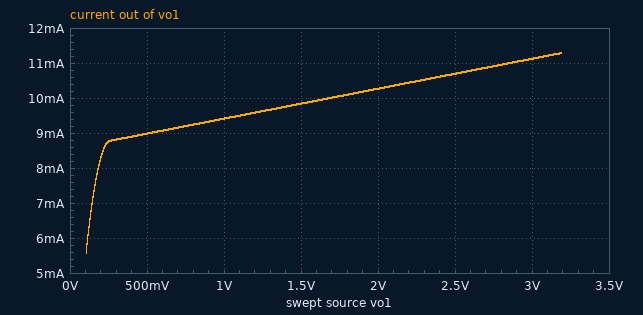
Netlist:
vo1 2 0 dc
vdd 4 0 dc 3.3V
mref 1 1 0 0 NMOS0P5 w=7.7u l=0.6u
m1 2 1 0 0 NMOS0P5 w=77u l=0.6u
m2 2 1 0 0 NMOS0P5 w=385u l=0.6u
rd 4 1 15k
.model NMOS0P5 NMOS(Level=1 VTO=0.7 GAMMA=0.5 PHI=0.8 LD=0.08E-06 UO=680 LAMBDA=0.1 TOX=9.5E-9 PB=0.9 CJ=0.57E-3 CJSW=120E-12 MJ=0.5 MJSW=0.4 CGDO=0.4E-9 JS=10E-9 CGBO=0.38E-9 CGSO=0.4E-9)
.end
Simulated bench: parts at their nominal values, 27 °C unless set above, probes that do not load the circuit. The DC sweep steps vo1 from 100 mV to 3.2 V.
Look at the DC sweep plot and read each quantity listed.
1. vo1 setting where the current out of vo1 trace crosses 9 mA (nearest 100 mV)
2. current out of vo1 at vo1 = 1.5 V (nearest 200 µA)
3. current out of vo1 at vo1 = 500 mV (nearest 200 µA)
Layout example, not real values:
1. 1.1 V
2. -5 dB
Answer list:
1. 500 mV
2. 9.8 mA
3. 9.0 mA
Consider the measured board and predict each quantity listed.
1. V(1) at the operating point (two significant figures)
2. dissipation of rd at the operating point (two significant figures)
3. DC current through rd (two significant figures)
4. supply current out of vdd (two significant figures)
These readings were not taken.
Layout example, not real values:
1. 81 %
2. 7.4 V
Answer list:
1. 960 mV
2. 370 µW
3. 160 µA
4. 160 µA
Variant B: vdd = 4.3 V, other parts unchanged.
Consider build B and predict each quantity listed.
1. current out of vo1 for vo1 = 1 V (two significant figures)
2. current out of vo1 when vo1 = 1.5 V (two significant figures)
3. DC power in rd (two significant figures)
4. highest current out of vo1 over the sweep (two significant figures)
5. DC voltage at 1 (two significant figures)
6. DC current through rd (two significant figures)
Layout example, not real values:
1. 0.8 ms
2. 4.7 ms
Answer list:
1. 13 mA
2. 14 mA
3. 720 µW
4. 16 mA
5. 1.0 V
6. 220 µA
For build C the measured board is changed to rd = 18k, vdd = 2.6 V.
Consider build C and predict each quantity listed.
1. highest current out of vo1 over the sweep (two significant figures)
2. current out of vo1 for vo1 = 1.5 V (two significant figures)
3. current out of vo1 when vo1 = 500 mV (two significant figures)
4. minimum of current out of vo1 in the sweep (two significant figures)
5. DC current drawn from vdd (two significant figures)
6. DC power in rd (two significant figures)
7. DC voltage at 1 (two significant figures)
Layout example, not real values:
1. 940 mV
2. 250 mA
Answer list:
1. 6.9 mA
2. 6.0 mA
3. 5.5 mA
4. 3.9 mA
5. 94 µA
6. 160 µW
7. 900 mV
